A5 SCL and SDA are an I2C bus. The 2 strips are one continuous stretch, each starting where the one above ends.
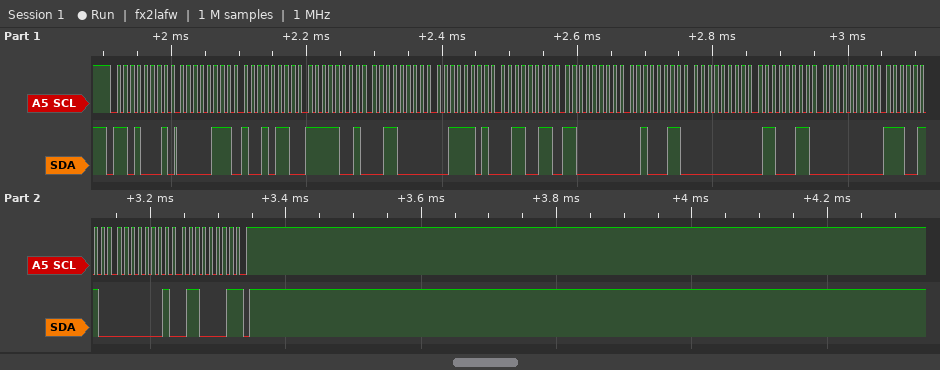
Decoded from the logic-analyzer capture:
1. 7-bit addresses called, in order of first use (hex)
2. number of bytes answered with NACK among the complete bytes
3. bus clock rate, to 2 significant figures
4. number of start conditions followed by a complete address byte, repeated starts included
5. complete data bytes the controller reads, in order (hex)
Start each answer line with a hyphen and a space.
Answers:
- 0x68
- 1
- 100 kHz
- 1
- 07 96 F9 30 3D 33 C0 23 00 63 00 E6 01 61
